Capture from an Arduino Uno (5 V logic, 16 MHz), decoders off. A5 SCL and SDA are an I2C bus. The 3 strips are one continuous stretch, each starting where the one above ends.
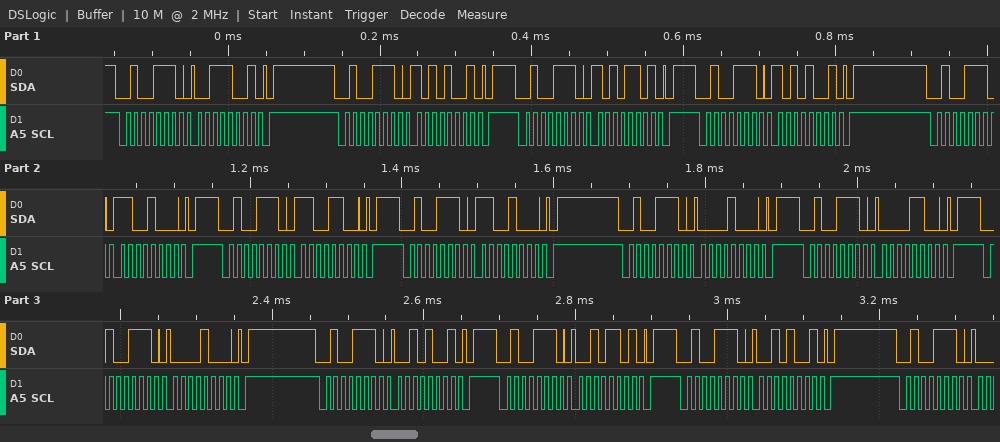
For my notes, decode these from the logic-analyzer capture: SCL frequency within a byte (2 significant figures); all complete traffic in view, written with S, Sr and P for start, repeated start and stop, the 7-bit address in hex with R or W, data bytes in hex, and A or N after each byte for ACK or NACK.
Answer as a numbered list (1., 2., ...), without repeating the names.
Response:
1. 100 kHz
2. S 27W A 39 A P S 27W A A9 A P S 27W A AD A P S 27W A A9 A P S 27W A C8 A P S 27W A CC A P S 27W A C8 A P S 27W A 08 A P S 27W A 0C A P S 27W A 08 A P S 27W A 29 A P S 27W A 2D A P S 27W A 29 A P S 27W A
